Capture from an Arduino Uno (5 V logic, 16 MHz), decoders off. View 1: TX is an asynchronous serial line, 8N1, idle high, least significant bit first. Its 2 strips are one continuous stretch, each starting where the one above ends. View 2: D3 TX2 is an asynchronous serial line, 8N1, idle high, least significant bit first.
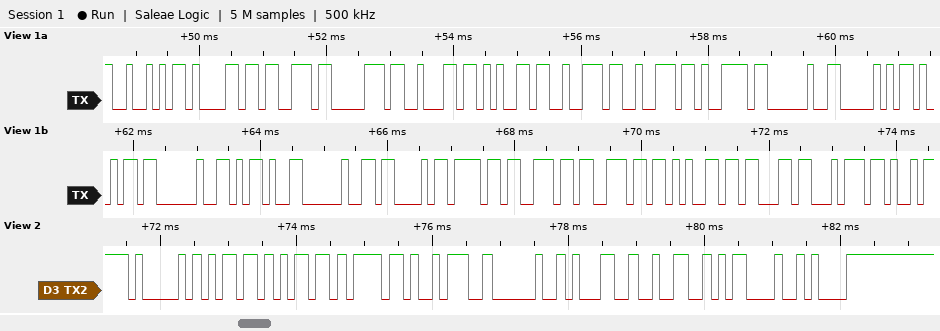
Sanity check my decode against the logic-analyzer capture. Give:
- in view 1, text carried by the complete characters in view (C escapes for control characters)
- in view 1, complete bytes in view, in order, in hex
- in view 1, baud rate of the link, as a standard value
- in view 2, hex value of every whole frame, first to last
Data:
"Raspberry Pi - Connect"
0x52 0x61 0x73 0x70 0x62 0x65 0x72 0x72 0x79 0x20 0x50 0x69 0x20 0x2D 0x20 0x43 0x6F 0x6E 0x6E 0x65 0x63 0x74
9600 baud
41 6D 6D 6F 3A 20 31 32 0D 0A
